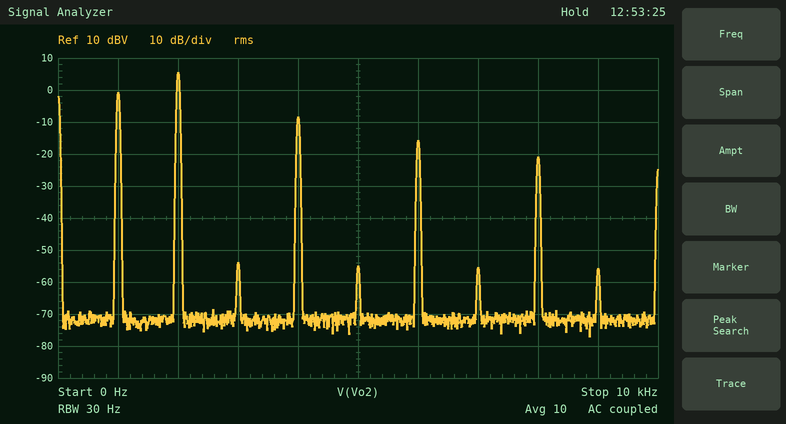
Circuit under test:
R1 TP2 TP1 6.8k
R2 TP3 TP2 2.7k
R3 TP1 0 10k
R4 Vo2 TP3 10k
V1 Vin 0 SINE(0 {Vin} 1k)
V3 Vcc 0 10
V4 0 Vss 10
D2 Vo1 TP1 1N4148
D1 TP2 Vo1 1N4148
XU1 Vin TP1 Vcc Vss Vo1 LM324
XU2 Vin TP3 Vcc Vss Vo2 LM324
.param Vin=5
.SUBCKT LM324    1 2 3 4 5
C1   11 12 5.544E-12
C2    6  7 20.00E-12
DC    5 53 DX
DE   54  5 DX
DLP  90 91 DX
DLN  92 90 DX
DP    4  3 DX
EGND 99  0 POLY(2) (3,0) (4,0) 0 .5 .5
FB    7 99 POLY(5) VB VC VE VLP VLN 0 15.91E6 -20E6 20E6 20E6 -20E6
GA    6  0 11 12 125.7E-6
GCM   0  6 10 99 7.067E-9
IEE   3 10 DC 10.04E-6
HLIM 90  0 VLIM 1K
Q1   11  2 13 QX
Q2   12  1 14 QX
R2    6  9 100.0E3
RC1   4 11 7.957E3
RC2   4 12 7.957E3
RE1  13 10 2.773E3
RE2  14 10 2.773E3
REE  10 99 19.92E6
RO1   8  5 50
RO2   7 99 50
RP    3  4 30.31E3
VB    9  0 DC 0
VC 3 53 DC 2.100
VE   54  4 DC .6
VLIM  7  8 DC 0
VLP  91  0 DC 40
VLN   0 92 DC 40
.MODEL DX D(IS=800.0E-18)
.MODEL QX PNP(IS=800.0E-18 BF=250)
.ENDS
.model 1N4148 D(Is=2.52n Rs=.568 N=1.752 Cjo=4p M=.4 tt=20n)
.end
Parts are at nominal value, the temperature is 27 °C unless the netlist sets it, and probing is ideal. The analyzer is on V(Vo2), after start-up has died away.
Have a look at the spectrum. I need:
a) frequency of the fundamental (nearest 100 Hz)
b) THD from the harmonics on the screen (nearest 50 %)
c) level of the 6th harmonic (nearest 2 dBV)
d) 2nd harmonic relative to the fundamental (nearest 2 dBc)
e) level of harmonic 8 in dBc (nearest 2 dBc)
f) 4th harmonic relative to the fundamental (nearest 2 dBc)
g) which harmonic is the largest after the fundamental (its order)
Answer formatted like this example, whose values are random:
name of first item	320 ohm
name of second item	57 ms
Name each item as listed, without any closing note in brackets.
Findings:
frequency of the fundamental	1.0 kHz
THD from the harmonics on the screen	200 %
level of the 6th harmonic	-16 dBV
2nd harmonic relative to the fundamental	6 dBc
level of harmonic 8 in dBc	-20 dBc
4th harmonic relative to the fundamental	-8 dBc
which harmonic is the largest after the fundamental	2
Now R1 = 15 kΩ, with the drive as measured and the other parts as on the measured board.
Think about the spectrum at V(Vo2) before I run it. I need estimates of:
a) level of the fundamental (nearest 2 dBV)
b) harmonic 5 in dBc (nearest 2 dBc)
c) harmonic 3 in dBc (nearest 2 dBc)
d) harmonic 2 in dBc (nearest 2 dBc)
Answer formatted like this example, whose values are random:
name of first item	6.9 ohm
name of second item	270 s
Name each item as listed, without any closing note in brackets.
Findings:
level of the fundamental	6 dBV
harmonic 5 in dBc	-14 dBc
harmonic 3 in dBc	-6 dBc
harmonic 2 in dBc	-2 dBc
